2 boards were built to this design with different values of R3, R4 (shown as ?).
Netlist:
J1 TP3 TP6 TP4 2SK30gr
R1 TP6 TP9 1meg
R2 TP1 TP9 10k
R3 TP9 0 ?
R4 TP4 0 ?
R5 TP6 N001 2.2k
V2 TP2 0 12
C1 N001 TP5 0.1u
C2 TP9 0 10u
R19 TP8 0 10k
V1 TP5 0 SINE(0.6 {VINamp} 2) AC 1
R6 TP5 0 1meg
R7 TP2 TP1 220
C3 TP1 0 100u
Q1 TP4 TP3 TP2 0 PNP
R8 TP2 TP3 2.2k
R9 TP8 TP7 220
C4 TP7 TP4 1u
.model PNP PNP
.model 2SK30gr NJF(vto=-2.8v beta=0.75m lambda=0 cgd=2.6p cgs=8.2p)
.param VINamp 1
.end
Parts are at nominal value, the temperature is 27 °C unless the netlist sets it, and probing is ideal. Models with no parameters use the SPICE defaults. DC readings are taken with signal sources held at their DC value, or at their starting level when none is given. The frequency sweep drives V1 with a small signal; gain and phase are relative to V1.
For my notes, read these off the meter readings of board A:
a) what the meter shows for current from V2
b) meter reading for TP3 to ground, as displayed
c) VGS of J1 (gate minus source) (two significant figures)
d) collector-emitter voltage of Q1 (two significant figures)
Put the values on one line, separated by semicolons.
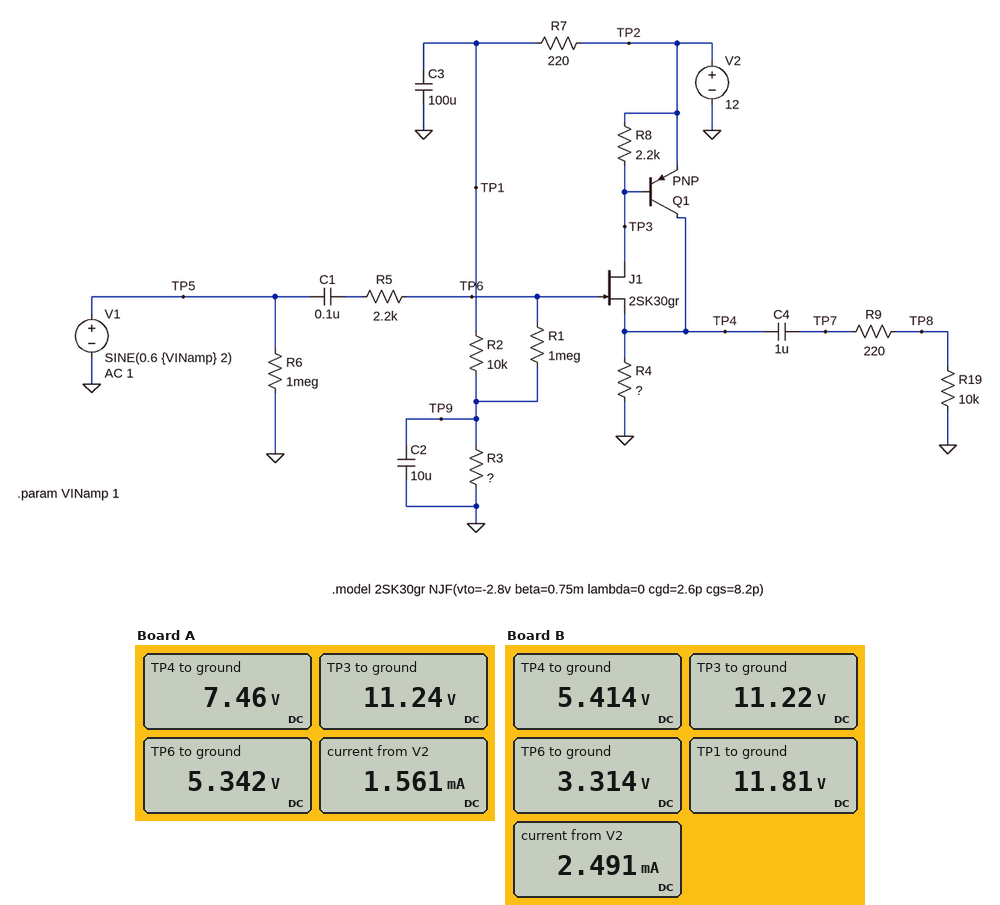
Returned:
1.561 mA; 11.24 V; -2.1 V; -4.5 V
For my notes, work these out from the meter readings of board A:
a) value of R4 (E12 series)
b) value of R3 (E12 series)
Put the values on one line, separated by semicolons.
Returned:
8.2 kΩ; 8.2 kΩ
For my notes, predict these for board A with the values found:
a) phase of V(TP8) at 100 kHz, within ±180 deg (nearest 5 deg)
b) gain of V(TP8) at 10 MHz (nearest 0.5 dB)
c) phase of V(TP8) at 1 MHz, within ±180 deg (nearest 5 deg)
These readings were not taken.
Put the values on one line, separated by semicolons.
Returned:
0 deg; 0 dB; 0 deg
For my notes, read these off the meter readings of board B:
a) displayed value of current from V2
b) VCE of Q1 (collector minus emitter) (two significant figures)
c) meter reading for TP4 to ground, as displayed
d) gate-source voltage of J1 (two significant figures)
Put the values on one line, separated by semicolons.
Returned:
2.491 mA; -6.6 V; 5.414 V; -2.1 V
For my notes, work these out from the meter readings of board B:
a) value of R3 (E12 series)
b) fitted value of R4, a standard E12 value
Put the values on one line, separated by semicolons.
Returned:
3.9 kΩ; 3.3 kΩ
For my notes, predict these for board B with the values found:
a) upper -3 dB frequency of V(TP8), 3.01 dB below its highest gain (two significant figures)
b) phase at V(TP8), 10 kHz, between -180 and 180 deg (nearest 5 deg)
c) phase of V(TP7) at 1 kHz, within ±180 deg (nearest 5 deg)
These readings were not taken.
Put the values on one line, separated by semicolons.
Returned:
65 MHz; 0 deg; 0 deg
